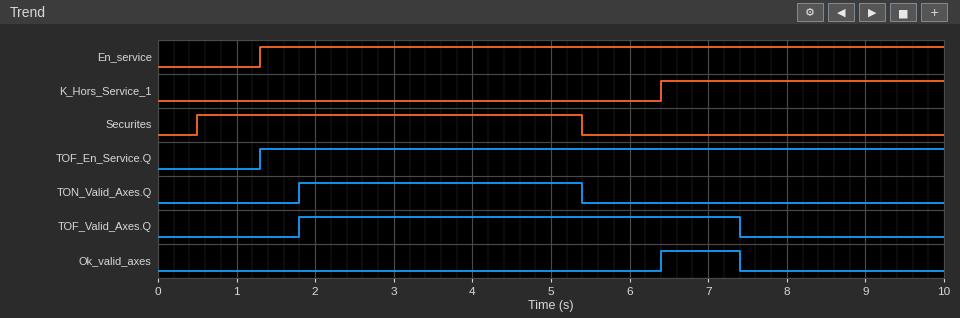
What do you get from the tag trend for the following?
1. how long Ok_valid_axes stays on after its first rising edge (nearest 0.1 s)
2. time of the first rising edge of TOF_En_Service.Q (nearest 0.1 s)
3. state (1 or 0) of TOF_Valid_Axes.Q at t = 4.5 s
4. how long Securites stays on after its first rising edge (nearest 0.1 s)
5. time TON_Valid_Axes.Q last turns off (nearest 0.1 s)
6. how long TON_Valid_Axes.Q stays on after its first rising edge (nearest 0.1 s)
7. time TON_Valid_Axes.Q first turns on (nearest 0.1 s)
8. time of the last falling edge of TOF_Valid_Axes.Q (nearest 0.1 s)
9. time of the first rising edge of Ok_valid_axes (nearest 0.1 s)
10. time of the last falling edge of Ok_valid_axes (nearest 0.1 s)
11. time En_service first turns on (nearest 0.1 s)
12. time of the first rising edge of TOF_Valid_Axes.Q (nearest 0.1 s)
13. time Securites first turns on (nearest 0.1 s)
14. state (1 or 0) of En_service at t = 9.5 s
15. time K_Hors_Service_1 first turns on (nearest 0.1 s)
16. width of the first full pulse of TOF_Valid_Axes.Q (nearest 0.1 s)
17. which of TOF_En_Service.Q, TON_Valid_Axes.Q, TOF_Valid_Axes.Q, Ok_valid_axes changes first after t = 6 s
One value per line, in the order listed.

1.0 s
1.3 s
1
4.9 s
5.4 s
3.6 s
1.8 s
7.4 s
6.4 s
7.4 s
1.3 s
1.8 s
0.5 s
1
6.4 s
5.6 s
Ok_valid_axes
